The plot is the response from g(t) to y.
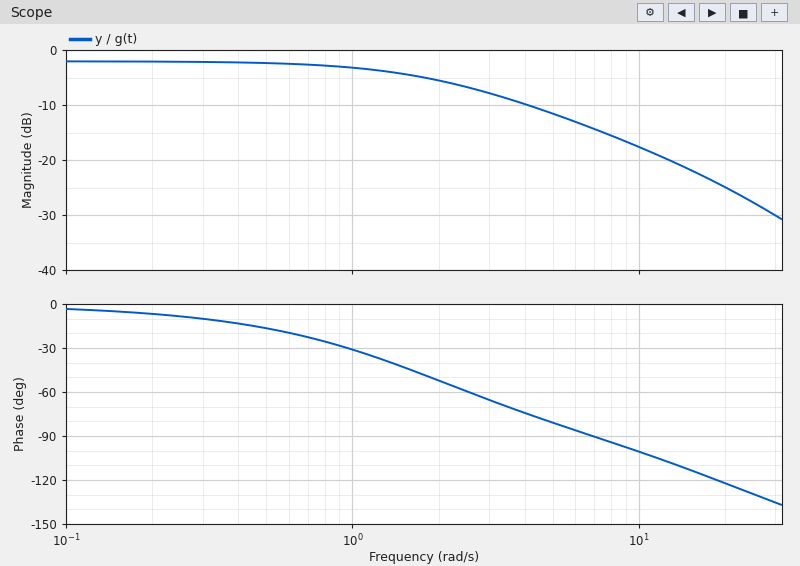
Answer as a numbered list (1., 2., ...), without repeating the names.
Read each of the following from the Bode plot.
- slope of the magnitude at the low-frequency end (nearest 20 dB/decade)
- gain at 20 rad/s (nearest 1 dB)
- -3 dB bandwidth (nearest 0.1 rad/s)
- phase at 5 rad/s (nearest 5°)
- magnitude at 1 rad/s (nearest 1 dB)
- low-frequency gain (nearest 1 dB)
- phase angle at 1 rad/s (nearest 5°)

1. 0 dB/decade
2. -25 dB
3. 1.8 rad/s
4. -80°
5. -3 dB
6. -2 dB
7. -30°
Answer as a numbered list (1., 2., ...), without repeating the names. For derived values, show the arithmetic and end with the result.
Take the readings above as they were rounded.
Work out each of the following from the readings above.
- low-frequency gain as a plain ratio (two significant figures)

1. 10^(-2 / 20) = 0.79
